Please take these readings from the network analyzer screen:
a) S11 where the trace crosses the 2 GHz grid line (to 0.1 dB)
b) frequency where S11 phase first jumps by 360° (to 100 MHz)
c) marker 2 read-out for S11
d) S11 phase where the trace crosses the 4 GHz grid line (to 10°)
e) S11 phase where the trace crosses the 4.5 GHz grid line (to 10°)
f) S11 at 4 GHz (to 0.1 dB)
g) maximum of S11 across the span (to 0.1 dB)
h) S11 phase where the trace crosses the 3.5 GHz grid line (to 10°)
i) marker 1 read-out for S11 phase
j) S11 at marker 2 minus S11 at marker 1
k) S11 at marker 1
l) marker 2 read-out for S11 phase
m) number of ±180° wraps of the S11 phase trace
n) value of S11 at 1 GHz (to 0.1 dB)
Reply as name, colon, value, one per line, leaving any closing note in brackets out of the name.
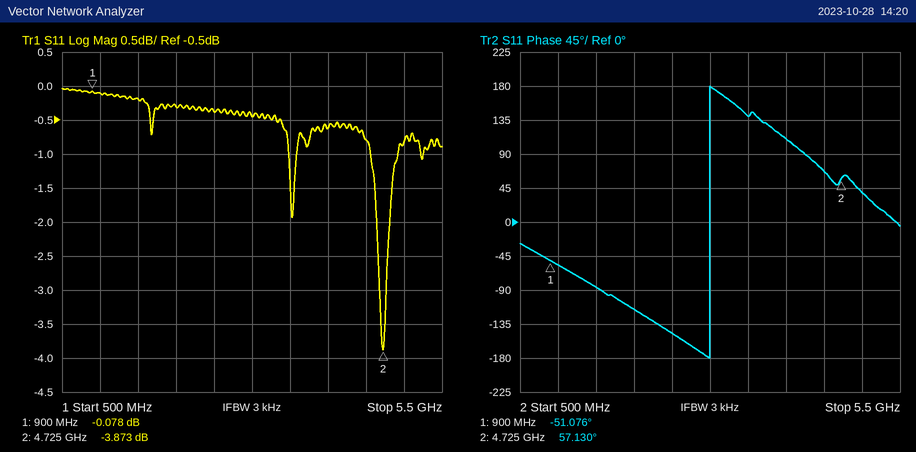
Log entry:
S11 where the trace crosses the 2 GHz grid line: -0.3 dB
frequency where S11 phase first jumps by 360°: 3.0 GHz
marker 2 read-out for S11: -3.873 dB
S11 phase where the trace crosses the 4 GHz grid line: 110°
S11 phase where the trace crosses the 4.5 GHz grid line: 70°
S11 at 4 GHz: -0.6 dB
maximum of S11 across the span: 0.0 dB
S11 phase where the trace crosses the 3.5 GHz grid line: 140°
marker 1 read-out for S11 phase: -51.076°
S11 at marker 2 minus S11 at marker 1: -3.795 dB
S11 at marker 1: -0.078 dB
marker 2 read-out for S11 phase: 57.130°
number of ±180° wraps of the S11 phase trace: 1
value of S11 at 1 GHz: -0.1 dB
